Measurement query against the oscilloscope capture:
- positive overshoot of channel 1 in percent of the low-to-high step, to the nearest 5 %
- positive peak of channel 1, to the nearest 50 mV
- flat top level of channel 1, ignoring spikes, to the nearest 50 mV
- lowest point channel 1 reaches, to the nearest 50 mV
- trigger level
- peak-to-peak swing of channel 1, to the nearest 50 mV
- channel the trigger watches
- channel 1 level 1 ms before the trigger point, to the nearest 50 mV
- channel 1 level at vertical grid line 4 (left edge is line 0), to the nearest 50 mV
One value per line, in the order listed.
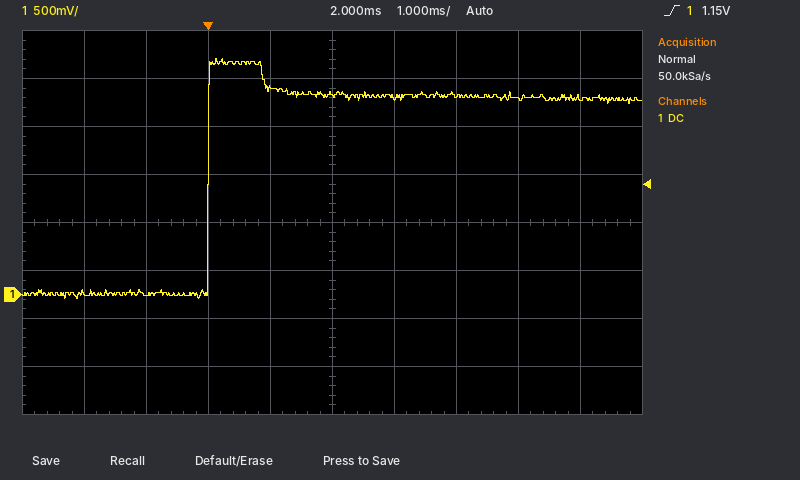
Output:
20 %
2.45 V
2.05 V
-50 mV
1.15 V
2.50 V
channel 1
0 mV
2.15 V
